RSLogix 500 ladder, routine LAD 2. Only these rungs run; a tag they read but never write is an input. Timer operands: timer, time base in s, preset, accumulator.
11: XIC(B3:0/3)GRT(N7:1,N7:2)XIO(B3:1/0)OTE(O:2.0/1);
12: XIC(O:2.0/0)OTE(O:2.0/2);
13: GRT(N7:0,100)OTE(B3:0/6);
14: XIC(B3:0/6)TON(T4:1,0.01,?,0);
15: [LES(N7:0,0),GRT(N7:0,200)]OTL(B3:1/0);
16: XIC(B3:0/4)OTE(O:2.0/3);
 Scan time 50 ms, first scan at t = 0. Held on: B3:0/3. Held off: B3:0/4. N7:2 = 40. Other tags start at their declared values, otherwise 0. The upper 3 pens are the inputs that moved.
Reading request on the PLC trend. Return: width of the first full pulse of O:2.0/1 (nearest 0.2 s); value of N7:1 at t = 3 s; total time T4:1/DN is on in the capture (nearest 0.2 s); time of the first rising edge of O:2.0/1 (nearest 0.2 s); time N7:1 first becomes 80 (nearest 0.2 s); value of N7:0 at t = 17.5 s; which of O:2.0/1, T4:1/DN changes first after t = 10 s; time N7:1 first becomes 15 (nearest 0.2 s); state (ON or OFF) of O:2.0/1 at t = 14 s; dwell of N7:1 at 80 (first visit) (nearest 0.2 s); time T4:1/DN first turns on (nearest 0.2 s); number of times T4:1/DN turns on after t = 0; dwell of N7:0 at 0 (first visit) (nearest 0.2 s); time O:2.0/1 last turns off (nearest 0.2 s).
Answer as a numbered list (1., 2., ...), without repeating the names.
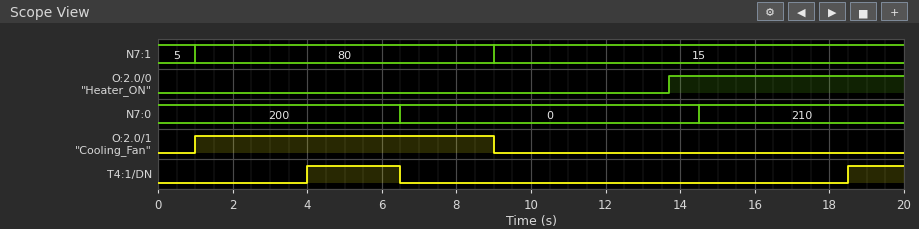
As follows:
1. 8.0 s
2. 80
3. 4.0 s
4. 1.0 s
5. 1.0 s
6. 210
7. T4:1/DN
8. 9.0 s
9. OFF
10. 8.0 s
11. 4.0 s
12. 2
13. 8.0 s
14. 9.0 s
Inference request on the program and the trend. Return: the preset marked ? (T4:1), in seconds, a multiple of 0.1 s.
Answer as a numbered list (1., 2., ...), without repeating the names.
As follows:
1. 4.0 s
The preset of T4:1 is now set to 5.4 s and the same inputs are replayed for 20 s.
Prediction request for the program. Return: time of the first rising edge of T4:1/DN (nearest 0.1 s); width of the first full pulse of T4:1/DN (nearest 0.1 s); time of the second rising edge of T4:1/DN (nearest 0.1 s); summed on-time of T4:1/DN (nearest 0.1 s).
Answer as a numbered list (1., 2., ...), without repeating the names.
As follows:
1. 5.4 s
2. 1.1 s
3. 19.9 s
4. 1.2 s
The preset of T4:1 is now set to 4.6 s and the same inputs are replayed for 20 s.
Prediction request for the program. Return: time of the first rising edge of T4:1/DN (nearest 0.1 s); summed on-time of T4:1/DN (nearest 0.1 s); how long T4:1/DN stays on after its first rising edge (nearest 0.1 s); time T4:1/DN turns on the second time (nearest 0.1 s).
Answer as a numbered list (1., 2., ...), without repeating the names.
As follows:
1. 4.6 s
2. 2.8 s
3. 1.9 s
4. 19.1 s
